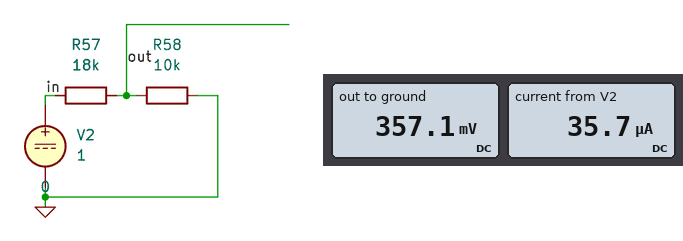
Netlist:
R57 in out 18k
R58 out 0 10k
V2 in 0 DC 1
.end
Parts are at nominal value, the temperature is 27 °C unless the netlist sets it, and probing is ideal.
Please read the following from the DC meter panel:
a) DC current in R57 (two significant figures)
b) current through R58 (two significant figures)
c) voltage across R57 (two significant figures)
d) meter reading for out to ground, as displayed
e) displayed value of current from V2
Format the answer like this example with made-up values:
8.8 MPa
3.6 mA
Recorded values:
36 µA
36 µA
640 mV
357.1 mV
35.7 µA
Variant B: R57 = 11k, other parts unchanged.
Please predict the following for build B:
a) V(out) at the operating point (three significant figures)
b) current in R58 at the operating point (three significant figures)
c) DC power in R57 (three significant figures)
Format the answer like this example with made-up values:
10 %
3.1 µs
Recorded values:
476 mV
47.6 µA
24.9 µW
